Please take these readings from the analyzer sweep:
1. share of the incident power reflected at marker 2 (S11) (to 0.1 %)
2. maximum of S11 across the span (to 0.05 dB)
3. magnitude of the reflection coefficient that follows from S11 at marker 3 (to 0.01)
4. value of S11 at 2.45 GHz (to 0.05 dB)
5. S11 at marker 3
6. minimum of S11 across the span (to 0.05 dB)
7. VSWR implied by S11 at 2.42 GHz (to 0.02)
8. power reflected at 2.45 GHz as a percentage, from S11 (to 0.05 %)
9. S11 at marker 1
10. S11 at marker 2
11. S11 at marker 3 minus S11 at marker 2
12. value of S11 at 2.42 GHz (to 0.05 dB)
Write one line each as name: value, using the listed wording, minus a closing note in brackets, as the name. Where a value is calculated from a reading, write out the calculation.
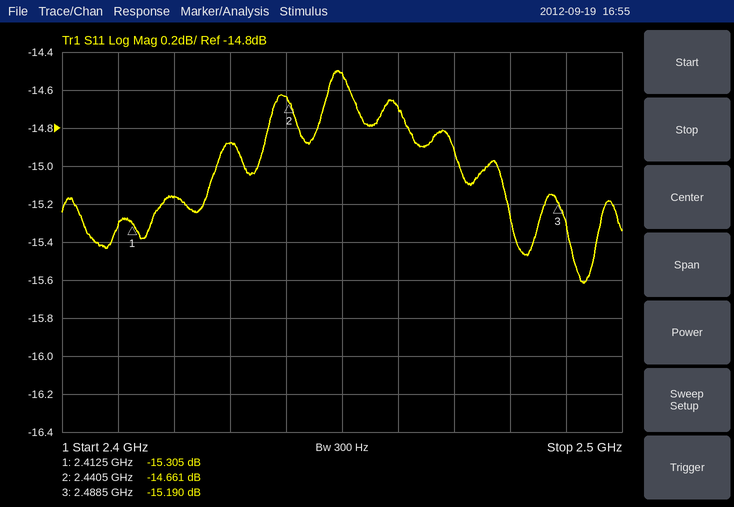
share of the incident power reflected at marker 2 (S11): 10^(-14.661/10) ≈ 3.4 %
maximum of S11 across the span: -14.50 dB
magnitude of the reflection coefficient that follows from S11 at marker 3: 10^(-15.19/20) ≈ 0.17
value of S11 at 2.45 GHz: -14.50 dB
S11 at marker 3: -15.190 dB
minimum of S11 across the span: -15.60 dB
VSWR implied by S11 at 2.42 GHz: |Γ| = 10^(-15.15/20) = 0.1748; VSWR = (1 + 0.1748)/(1 − 0.1748) ≈ 1.42
power reflected at 2.45 GHz as a percentage, from S11: 10^(-14.5/10) ≈ 3.55 %
S11 at marker 1: -15.305 dB
S11 at marker 2: -14.661 dB
S11 at marker 3 minus S11 at marker 2: -15.19 − (-14.661) = -0.529 dB
value of S11 at 2.42 GHz: -15.15 dB
